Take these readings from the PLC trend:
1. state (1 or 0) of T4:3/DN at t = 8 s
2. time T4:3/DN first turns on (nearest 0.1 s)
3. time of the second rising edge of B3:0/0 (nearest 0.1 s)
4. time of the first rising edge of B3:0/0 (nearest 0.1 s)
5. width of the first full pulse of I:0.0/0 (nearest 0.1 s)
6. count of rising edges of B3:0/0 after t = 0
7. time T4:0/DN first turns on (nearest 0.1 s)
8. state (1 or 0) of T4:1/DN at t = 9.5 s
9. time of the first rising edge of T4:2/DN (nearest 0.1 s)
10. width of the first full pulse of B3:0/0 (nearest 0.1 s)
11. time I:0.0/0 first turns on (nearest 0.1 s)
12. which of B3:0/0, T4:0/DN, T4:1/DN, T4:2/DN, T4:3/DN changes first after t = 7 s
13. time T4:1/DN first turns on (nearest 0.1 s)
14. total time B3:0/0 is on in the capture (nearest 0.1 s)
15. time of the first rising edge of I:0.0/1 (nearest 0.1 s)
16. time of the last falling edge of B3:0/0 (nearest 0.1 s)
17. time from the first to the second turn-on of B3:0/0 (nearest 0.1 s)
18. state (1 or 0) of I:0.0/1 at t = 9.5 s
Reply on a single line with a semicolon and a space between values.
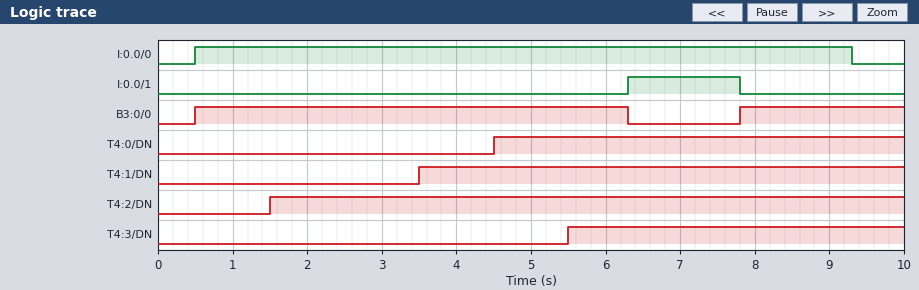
1; 5.5 s; 7.8 s; 0.5 s; 8.8 s; 2; 4.5 s; 1; 1.5 s; 5.8 s; 0.5 s; B3:0/0; 3.5 s; 8.0 s; 6.3 s; 6.3 s; 7.3 s; 0
